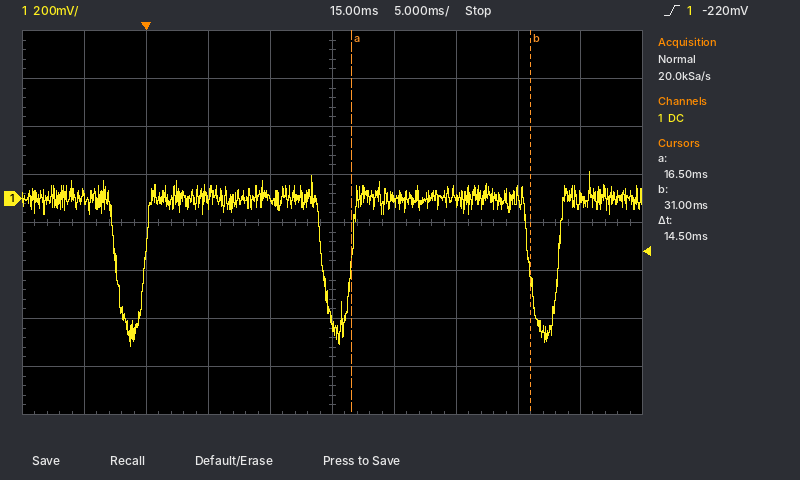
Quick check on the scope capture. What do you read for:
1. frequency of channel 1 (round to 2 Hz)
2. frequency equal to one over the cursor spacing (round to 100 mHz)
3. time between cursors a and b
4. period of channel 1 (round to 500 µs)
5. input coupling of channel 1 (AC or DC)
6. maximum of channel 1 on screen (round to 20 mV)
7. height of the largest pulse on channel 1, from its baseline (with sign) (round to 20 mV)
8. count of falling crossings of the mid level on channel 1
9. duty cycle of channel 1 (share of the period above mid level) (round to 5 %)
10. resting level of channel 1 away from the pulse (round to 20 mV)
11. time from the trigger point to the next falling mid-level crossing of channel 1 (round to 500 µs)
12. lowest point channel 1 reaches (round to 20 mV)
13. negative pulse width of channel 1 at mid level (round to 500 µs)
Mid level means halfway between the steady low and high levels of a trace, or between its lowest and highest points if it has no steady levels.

60 Hz
69.0 Hz
14.5 ms
16.5 ms
DC
120 mV
-620 mV
3
85 %
0 mV
14.0 ms
-620 mV
2.5 ms
